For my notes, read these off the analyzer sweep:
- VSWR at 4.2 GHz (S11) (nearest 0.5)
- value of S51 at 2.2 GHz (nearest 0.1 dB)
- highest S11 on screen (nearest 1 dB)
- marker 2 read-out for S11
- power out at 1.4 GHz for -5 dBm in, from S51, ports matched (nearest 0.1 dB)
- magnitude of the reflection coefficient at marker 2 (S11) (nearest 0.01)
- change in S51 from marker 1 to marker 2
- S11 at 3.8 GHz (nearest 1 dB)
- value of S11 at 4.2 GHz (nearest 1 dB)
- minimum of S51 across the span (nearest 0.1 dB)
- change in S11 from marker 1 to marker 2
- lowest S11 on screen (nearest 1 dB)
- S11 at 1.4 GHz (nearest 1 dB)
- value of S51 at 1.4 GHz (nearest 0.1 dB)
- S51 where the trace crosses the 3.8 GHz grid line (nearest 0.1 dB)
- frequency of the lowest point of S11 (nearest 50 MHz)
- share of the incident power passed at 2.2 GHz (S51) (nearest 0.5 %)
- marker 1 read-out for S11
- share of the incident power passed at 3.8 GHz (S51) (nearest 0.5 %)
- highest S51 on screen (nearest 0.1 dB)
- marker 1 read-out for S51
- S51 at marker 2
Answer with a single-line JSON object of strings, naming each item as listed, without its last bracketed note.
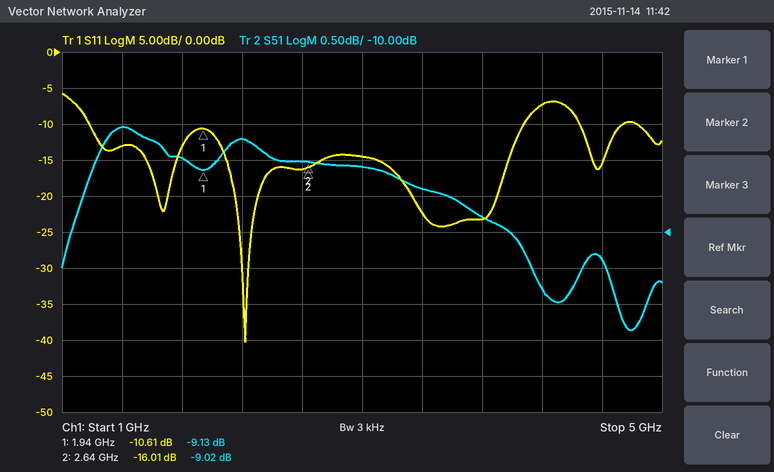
{"VSWR at 4.2 GHz (S11)": "2.5", "value of S51 at 2.2 GHz": "-8.7 dB", "highest S11 on screen": "-6 dB", "marker 2 read-out for S11": "-16.01 dB", "power out at 1.4 GHz for -5 dBm in, from S51, ports matched": "-13.5 dBm", "magnitude of the reflection coefficient at marker 2 (S11)": "0.16", "change in S51 from marker 1 to marker 2": "0.11 dB", "S11 at 3.8 GHz": "-23 dB", "value of S11 at 4.2 GHz": "-7 dB", "minimum of S51 across the span": "-11.4 dB", "change in S11 from marker 1 to marker 2": "-5.40 dB", "lowest S11 on screen": "-40 dB", "S11 at 1.4 GHz": "-13 dB", "value of S51 at 1.4 GHz": "-8.5 dB", "S51 where the trace crosses the 3.8 GHz grid line": "-9.8 dB", "frequency of the lowest point of S11": "2.20 GHz", "share of the incident power passed at 2.2 GHz (S51)": "13.5 %", "marker 1 read-out for S11": "-10.61 dB", "share of the incident power passed at 3.8 GHz (S51)": "10.5 %", "highest S51 on screen": "-8.5 dB", "marker 1 read-out for S51": "-9.13 dB", "S51 at marker 2": "-9.02 dB"}
